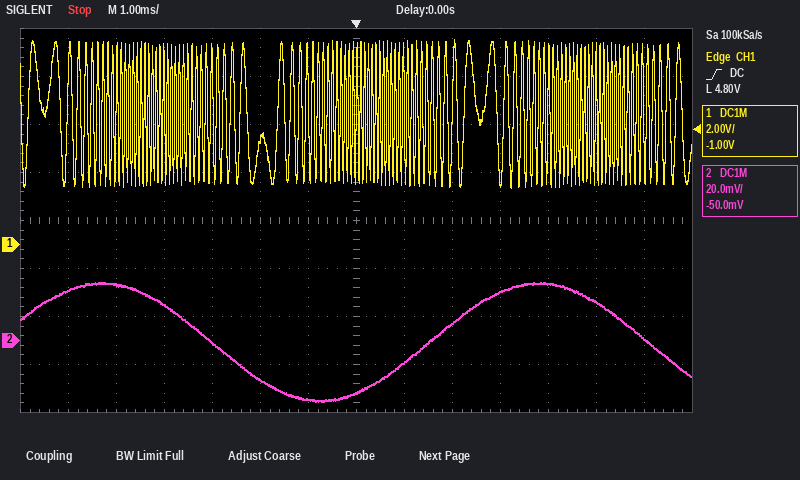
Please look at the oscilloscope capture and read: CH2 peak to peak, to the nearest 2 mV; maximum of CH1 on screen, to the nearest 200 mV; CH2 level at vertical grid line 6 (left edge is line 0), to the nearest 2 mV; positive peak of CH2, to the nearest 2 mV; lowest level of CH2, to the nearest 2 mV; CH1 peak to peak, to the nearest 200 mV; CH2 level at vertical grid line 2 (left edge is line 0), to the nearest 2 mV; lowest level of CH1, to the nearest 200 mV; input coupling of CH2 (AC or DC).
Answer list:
50 mV
8.6 V
-24 mV
24 mV
-26 mV
6.2 V
24 mV
2.4 V
DC
